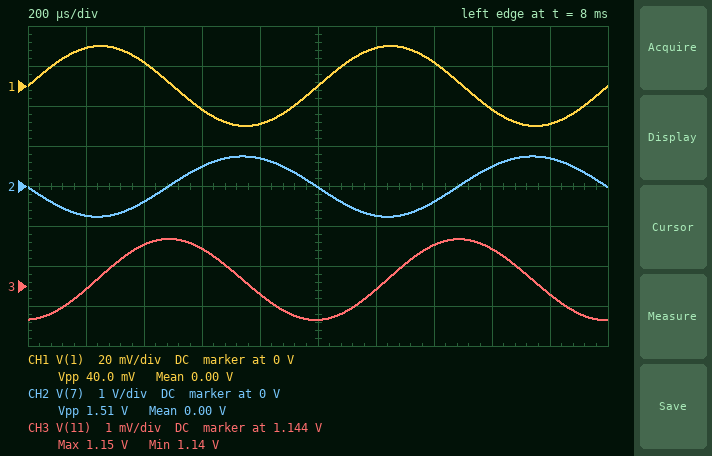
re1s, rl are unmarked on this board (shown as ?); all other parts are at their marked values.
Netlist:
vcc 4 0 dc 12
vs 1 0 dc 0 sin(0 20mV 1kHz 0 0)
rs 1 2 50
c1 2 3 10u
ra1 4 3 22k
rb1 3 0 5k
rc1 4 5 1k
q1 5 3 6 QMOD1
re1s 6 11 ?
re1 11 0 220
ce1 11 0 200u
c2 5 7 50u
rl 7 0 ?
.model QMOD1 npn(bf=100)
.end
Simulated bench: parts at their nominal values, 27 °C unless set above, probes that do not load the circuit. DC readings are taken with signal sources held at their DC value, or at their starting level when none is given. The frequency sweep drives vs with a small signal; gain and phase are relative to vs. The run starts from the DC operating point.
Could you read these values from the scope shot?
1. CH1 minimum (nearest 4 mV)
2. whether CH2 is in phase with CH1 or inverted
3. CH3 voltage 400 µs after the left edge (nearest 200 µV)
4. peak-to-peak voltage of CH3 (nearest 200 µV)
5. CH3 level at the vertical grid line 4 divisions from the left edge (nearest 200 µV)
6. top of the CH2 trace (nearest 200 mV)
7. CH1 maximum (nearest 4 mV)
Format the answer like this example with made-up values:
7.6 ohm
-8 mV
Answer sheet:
-20 mV
inverted
1.1450 V
2.0 mV
1.1438 V
800 mV
20 mV
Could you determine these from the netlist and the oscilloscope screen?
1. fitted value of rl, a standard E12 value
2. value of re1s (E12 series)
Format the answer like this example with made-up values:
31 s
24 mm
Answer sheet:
1.5 kΩ
10 Ω
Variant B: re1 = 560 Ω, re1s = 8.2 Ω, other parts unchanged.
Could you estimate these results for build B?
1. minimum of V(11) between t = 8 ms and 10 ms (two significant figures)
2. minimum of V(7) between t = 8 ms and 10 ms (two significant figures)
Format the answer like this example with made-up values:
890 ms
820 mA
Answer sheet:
1.3 V
-620 mV
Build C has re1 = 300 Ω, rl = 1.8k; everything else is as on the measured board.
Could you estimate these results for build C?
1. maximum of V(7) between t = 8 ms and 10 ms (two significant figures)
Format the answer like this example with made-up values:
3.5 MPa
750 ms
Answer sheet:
720 mV
